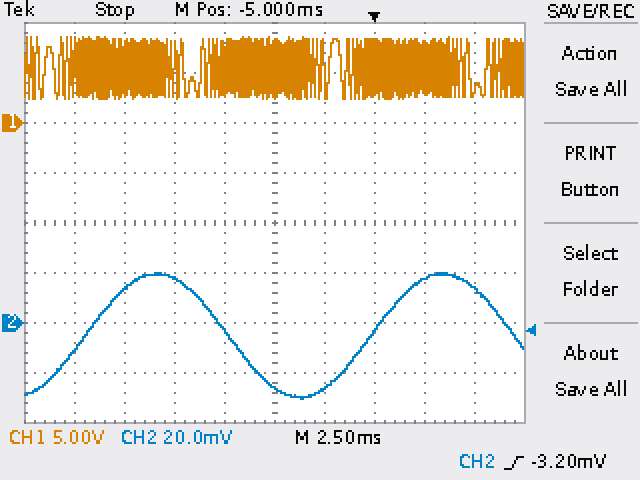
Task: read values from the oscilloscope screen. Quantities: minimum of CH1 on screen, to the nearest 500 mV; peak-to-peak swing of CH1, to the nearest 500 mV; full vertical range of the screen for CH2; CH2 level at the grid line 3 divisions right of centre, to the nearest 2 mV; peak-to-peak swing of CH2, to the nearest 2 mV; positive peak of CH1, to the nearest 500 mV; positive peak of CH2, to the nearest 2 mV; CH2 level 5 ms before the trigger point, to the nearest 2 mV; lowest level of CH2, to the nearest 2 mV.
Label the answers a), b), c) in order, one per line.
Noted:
a) 2.5 V
b) 6.0 V
c) 160 mV
d) 18 mV
e) 50 mV
f) 8.5 V
g) 20 mV
h) -26 mV
i) -30 mV
